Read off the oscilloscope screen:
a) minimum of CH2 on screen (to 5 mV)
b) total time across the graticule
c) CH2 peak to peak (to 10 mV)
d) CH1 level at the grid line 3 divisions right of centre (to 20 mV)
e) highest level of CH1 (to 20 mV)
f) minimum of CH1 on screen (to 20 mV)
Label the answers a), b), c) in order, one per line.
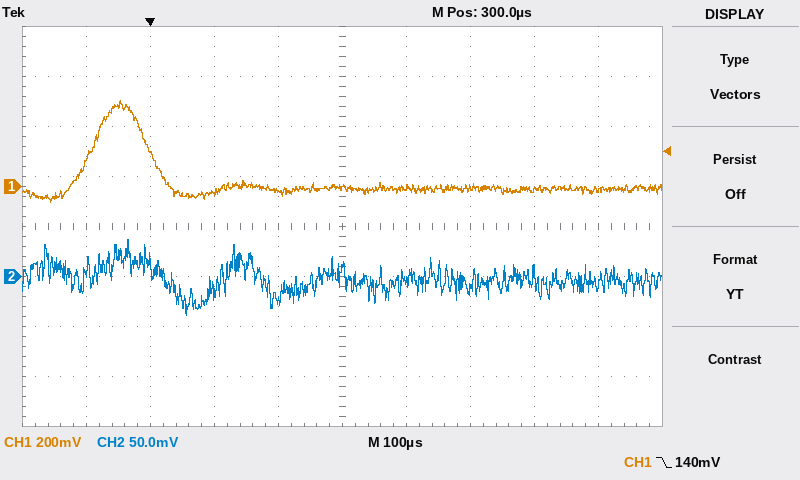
a) -40 mV
b) 1 ms
c) 80 mV
d) -20 mV
e) 340 mV
f) -60 mV
